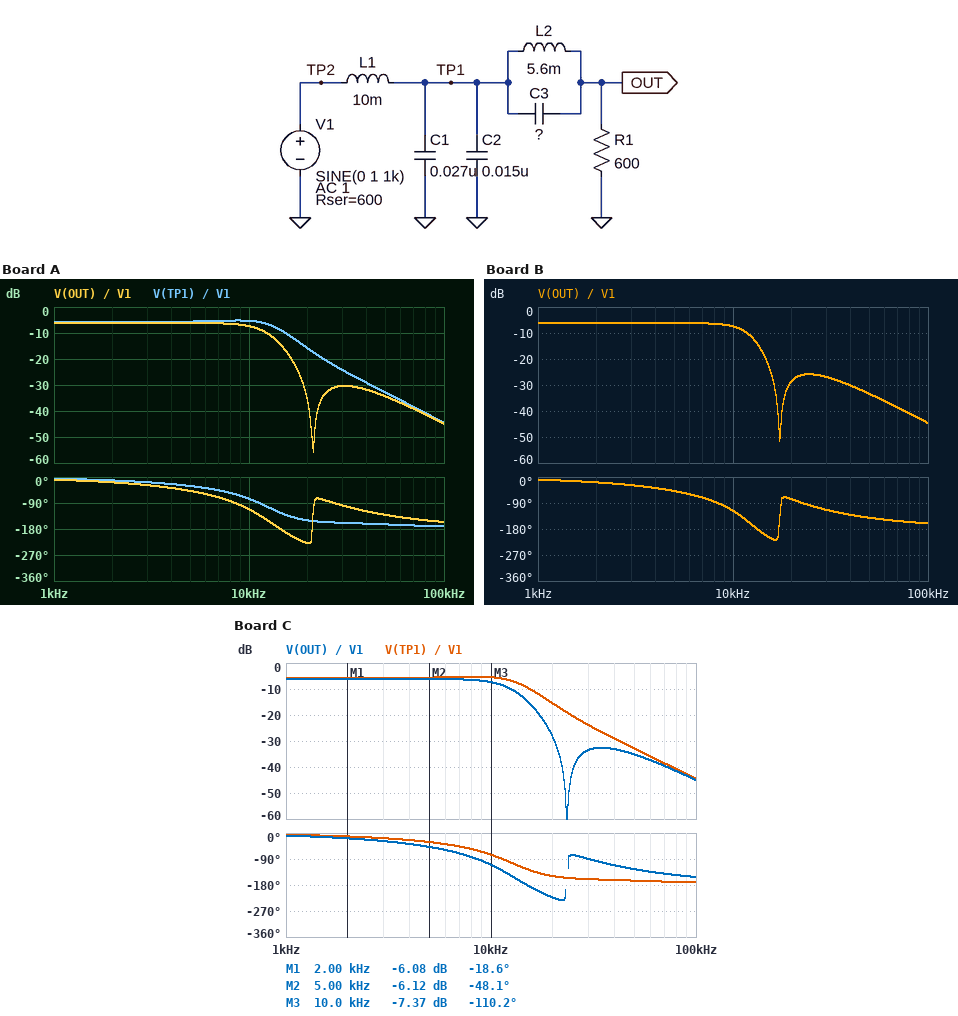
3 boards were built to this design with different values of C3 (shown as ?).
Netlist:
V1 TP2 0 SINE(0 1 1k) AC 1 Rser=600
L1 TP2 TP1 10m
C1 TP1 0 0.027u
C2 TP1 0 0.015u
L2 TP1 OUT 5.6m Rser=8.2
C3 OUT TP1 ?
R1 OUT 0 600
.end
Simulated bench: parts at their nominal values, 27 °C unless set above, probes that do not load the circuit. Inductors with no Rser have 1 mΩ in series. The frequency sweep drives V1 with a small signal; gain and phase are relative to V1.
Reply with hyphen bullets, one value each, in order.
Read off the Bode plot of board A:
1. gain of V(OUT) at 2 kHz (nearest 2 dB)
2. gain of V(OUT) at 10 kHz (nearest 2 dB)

- -6 dB
- -8 dB
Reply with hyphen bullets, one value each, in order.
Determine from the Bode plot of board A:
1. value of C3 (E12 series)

- 10 nF
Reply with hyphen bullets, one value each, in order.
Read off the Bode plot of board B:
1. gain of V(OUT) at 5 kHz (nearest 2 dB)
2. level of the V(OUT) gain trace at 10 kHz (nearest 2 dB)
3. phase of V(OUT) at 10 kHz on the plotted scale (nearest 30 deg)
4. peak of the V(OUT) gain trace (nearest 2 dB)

- -6 dB
- -8 dB
- -120 deg
- -6 dB
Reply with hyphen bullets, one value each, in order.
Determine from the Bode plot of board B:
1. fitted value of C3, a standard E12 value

- 15 nF
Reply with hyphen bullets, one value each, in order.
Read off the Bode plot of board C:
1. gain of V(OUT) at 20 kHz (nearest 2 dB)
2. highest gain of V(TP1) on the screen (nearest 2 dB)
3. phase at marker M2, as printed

- -28 dB
- -6 dB
- -48.1 deg
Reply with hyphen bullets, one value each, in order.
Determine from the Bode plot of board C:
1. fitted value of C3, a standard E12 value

- 8.2 nF
